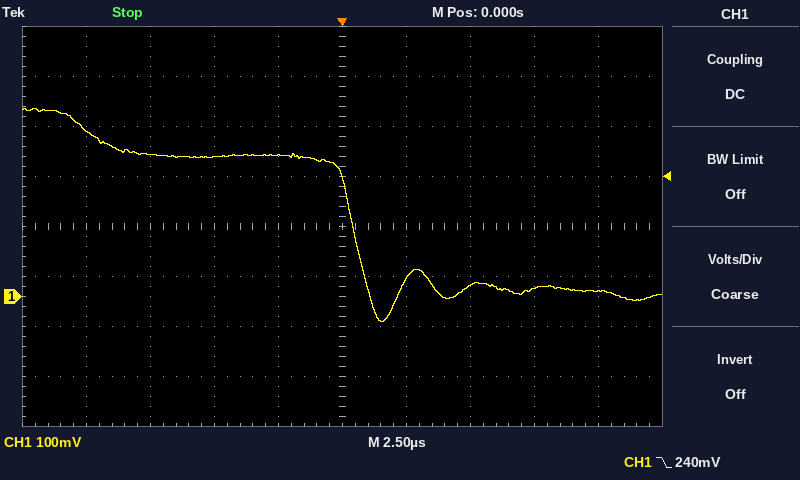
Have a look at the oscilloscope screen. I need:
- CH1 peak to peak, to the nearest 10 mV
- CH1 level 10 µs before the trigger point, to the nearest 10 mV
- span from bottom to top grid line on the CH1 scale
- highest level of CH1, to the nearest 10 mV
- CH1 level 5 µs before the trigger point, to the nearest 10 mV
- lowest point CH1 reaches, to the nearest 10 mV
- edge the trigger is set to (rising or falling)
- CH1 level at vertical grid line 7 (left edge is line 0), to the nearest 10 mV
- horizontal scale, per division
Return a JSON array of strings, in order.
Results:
["430 mV", "330 mV", "800 mV", "380 mV", "280 mV", "-50 mV", "falling", "20 mV", "2.5 µs"]
